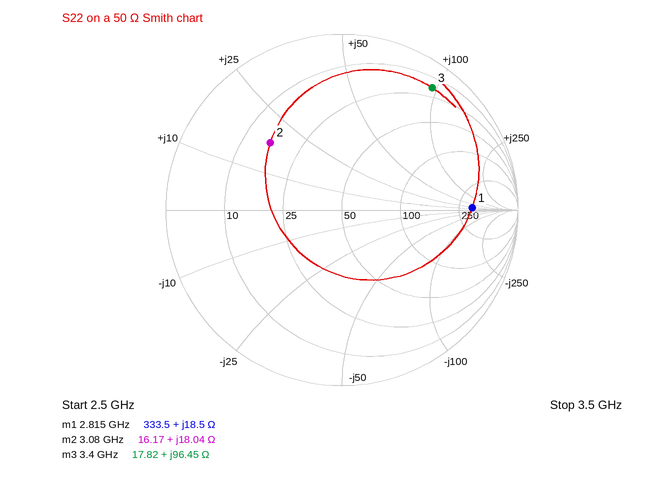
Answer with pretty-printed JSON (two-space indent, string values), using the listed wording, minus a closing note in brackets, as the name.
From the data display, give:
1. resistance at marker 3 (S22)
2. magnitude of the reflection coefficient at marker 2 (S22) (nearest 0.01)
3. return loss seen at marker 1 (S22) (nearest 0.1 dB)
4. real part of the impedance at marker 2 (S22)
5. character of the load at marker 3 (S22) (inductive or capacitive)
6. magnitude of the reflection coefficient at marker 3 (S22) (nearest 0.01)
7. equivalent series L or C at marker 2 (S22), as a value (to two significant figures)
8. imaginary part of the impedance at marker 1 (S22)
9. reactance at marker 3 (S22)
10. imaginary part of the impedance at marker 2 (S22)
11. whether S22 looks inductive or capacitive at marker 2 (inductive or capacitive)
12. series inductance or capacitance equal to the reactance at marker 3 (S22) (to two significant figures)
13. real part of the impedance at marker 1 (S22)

{
  "resistance at marker 3": "17.82 Ω",
  "magnitude of the reflection coefficient at marker 2 (S22)": "0.56",
  "return loss seen at marker 1 (S22)": "2.6 dB",
  "real part of the impedance at marker 2": "16.17 Ω",
  "character of the load at marker 3 (S22)": "inductive",
  "magnitude of the reflection coefficient at marker 3 (S22)": "0.86",
  "equivalent series L or C at marker 2 (S22), as a value": "930 pH",
  "imaginary part of the impedance at marker 1": "+18.5 Ω",
  "reactance at marker 3": "+96.45 Ω",
  "imaginary part of the impedance at marker 2": "+18.04 Ω",
  "whether S22 looks inductive or capacitive at marker 2": "inductive",
  "series inductance or capacitance equal to the reactance at marker 3 (S22)": "4.5 nH",
  "real part of the impedance at marker 1": "333.5 Ω"
}
